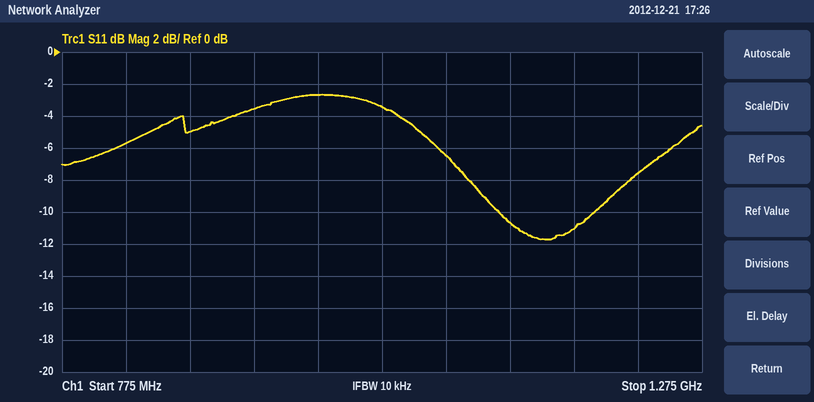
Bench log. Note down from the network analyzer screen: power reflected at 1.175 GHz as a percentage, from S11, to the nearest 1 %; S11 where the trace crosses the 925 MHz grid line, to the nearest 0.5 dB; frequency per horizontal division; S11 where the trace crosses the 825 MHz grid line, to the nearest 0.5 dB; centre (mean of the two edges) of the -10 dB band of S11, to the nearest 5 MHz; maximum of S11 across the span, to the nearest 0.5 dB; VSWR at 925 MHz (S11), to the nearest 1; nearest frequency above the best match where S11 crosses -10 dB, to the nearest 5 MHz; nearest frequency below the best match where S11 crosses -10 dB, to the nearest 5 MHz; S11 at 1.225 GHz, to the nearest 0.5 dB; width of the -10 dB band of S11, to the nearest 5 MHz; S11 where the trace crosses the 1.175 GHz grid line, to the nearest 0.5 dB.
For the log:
8 %
-3.5 dB
50 MHz
-5.5 dB
1.155 GHz
-2.5 dB
5
1.190 GHz
1.115 GHz
-7.5 dB
75 MHz
-11.0 dB
